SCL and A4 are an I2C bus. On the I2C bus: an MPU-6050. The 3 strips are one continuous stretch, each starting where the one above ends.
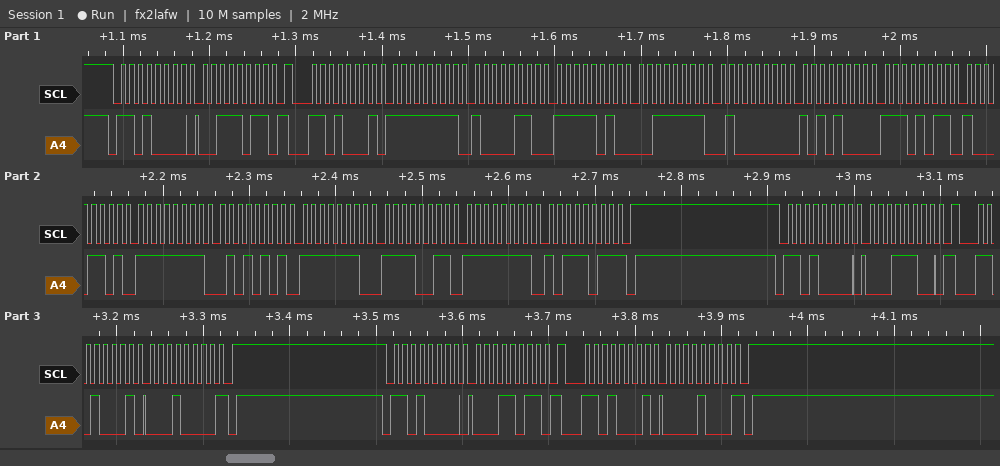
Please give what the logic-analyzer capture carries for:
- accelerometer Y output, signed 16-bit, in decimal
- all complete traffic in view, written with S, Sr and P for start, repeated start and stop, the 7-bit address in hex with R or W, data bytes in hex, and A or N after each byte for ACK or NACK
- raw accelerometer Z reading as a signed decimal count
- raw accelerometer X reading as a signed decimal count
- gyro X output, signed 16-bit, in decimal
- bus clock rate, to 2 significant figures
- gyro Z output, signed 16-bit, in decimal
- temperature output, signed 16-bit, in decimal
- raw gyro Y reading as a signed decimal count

-1473
S 68W A 3B A Sr 68R A FF A 86 A FA A 3F A 40 A A8 A EB A 8D A FF A 55 A FE A F3 A FF A BB N P S 68W A 1C A Sr 68R A 10 N P S 68W A 1B A Sr 68R A 08 N P
16552
-122
-171
100 kHz
-69
-5235
-269
